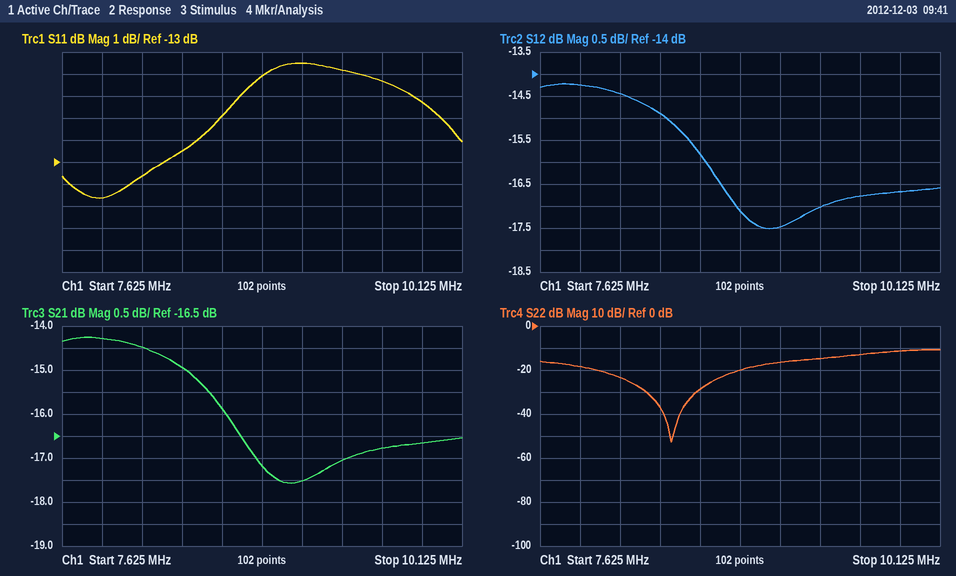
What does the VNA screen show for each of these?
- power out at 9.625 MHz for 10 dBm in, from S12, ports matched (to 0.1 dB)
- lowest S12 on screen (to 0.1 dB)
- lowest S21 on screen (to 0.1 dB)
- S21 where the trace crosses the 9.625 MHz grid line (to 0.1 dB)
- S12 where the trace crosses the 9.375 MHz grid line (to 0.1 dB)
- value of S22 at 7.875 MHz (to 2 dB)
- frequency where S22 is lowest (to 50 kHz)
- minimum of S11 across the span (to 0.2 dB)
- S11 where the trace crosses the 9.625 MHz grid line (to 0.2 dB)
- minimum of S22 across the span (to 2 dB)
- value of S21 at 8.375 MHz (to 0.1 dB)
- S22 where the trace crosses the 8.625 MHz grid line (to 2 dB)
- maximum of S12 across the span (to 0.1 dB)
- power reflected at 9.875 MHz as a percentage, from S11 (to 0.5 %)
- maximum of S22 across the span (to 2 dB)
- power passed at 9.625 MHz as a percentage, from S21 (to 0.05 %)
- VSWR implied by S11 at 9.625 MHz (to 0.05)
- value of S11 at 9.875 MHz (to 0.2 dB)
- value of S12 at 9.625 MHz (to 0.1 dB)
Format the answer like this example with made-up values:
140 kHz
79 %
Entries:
-6.8 dBm
-17.5 dB
-17.6 dB
-16.8 dB
-17.0 dB
-18 dB
8.45 MHz
-14.6 dB
-9.4 dB
-52 dB
-14.9 dB
-28 dB
-14.2 dB
9.5 %
-10 dB
2.10 %
2.05
-10.2 dB
-16.8 dB
